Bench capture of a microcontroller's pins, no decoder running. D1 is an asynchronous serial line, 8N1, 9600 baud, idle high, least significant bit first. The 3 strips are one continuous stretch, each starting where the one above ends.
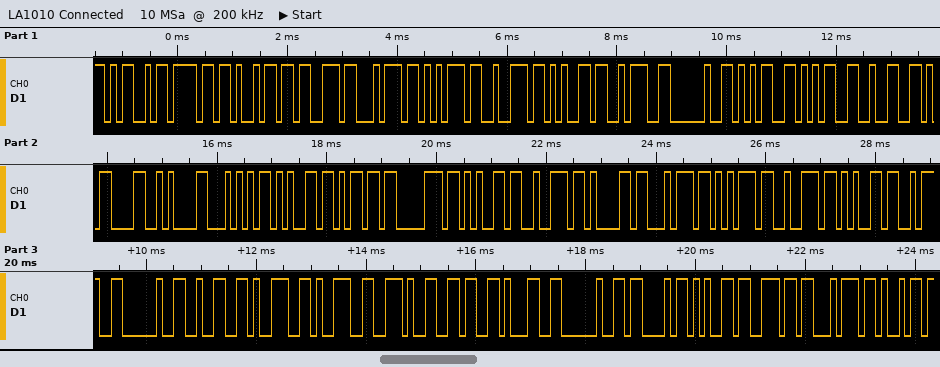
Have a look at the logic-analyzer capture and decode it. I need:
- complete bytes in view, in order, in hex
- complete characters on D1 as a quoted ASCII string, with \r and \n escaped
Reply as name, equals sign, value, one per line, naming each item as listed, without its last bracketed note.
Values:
complete bytes in view, in order, in hex = 4D 6F 69 73 74 75 72 65 3A 20 35 35 32 0D 0A 54 65 6D 70 65 72 61 74 75 72 65 3A 20 32 39 39 2E 36 31 20 43 65 6E 74 69
complete characters on D1 as a quoted ASCII string, with \r and \n escaped = "Moisture: 552\r\nTemperature: 299.61 Centi"
